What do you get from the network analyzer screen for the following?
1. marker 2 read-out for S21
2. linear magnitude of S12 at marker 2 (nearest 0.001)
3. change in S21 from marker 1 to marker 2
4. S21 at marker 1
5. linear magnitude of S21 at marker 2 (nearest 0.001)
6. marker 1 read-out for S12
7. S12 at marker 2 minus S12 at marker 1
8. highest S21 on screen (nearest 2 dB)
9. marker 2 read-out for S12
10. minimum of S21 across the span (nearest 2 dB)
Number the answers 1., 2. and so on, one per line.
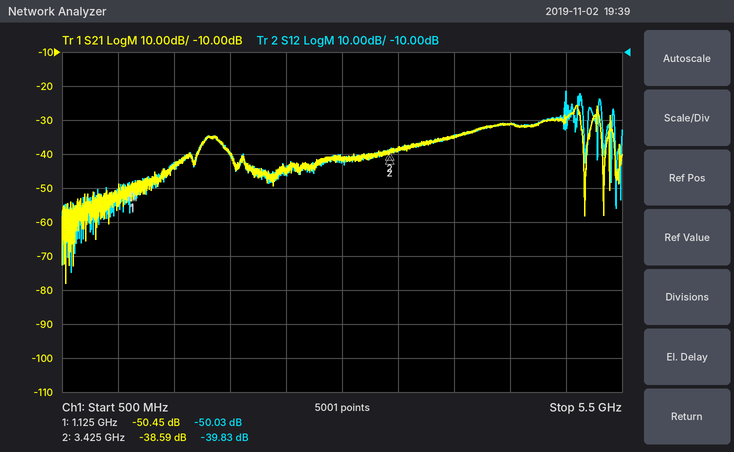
1. -38.59 dB
2. 0.010
3. 11.86 dB
4. -50.45 dB
5. 0.012
6. -50.03 dB
7. 10.20 dB
8. -26 dB
9. -39.83 dB
10. -78 dB
